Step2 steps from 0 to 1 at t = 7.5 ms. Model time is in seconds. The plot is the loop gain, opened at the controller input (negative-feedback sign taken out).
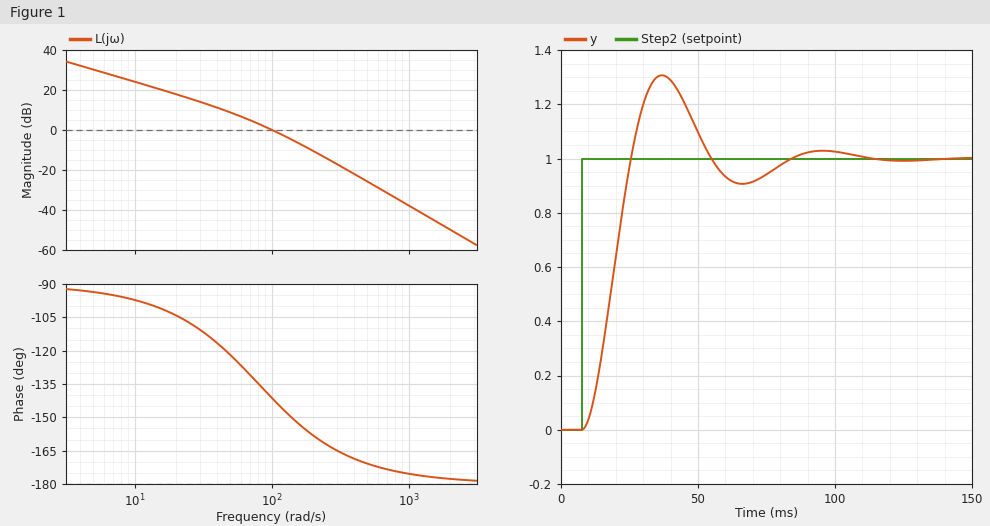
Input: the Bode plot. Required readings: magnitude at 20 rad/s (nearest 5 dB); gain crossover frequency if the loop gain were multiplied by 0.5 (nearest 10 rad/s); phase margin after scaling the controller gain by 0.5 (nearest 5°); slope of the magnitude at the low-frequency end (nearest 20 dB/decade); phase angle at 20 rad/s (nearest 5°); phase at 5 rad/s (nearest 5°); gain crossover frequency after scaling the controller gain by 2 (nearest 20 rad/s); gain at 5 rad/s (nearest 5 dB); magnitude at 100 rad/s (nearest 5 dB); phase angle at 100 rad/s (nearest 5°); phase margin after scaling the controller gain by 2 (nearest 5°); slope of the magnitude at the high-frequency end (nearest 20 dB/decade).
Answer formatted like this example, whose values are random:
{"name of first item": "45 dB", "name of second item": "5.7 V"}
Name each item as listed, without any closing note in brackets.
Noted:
{"magnitude at 20 rad/s": "20 dB", "gain crossover frequency if the loop gain were multiplied by 0.5": "60 rad/s", "phase margin after scaling the controller gain by 0.5": "50°", "slope of the magnitude at the low-frequency end": "-20 dB/decade", "phase angle at 20 rad/s": "-105°", "phase at 5 rad/s": "-95°", "gain crossover frequency after scaling the controller gain by 2": "160 rad/s", "gain at 5 rad/s": "30 dB", "magnitude at 100 rad/s": "0 dB", "phase angle at 100 rad/s": "-140°", "phase margin after scaling the controller gain by 2": "30°", "slope of the magnitude at the high-frequency end": "-40 dB/decade"}
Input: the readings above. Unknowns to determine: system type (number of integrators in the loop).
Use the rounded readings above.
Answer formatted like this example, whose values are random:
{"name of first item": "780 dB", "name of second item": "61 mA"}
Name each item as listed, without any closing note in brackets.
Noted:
{"system type": "1"}
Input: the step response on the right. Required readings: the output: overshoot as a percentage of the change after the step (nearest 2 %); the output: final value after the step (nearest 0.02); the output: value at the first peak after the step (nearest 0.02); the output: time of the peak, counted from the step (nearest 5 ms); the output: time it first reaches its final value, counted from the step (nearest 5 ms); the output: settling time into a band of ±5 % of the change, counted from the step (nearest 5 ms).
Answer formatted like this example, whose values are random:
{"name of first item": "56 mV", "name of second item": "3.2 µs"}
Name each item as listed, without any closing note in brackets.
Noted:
{"the output: overshoot as a percentage of the change after the step": "30 %", "the output: final value after the step": "1.00", "the output: value at the first peak after the step": "1.30", "the output: time of the peak, counted from the step": "30 ms", "the output: time it first reaches its final value, counted from the step": "20 ms", "the output: settling time into a band of ±5 % of the change, counted from the step": "70 ms"}
